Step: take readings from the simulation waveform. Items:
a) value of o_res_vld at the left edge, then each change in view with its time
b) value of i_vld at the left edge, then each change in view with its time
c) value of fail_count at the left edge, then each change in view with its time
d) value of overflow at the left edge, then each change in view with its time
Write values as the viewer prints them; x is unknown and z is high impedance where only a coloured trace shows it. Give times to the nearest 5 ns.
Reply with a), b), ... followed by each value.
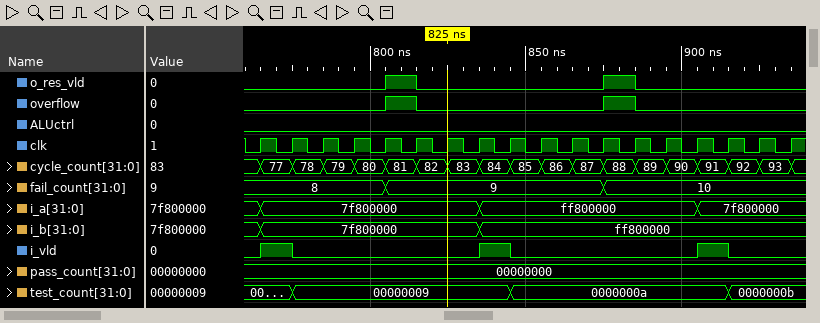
a) 0, 1 at 805 ns, 0 at 815 ns, 1 at 875 ns, 0 at 885 ns
b) 0, 1 at 765 ns, 0 at 775 ns, 1 at 835 ns, 0 at 845 ns, 1 at 905 ns, 0 at 915 ns
c) 8, 9 at 805 ns, 10 at 875 ns
d) 0, 1 at 805 ns, 0 at 815 ns, 1 at 875 ns, 0 at 885 ns
